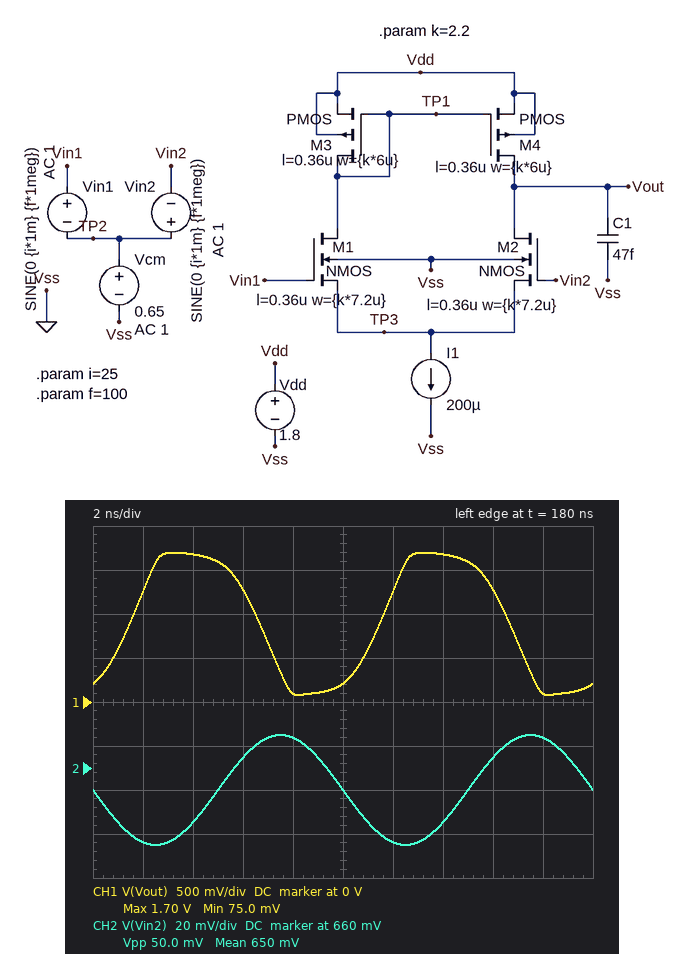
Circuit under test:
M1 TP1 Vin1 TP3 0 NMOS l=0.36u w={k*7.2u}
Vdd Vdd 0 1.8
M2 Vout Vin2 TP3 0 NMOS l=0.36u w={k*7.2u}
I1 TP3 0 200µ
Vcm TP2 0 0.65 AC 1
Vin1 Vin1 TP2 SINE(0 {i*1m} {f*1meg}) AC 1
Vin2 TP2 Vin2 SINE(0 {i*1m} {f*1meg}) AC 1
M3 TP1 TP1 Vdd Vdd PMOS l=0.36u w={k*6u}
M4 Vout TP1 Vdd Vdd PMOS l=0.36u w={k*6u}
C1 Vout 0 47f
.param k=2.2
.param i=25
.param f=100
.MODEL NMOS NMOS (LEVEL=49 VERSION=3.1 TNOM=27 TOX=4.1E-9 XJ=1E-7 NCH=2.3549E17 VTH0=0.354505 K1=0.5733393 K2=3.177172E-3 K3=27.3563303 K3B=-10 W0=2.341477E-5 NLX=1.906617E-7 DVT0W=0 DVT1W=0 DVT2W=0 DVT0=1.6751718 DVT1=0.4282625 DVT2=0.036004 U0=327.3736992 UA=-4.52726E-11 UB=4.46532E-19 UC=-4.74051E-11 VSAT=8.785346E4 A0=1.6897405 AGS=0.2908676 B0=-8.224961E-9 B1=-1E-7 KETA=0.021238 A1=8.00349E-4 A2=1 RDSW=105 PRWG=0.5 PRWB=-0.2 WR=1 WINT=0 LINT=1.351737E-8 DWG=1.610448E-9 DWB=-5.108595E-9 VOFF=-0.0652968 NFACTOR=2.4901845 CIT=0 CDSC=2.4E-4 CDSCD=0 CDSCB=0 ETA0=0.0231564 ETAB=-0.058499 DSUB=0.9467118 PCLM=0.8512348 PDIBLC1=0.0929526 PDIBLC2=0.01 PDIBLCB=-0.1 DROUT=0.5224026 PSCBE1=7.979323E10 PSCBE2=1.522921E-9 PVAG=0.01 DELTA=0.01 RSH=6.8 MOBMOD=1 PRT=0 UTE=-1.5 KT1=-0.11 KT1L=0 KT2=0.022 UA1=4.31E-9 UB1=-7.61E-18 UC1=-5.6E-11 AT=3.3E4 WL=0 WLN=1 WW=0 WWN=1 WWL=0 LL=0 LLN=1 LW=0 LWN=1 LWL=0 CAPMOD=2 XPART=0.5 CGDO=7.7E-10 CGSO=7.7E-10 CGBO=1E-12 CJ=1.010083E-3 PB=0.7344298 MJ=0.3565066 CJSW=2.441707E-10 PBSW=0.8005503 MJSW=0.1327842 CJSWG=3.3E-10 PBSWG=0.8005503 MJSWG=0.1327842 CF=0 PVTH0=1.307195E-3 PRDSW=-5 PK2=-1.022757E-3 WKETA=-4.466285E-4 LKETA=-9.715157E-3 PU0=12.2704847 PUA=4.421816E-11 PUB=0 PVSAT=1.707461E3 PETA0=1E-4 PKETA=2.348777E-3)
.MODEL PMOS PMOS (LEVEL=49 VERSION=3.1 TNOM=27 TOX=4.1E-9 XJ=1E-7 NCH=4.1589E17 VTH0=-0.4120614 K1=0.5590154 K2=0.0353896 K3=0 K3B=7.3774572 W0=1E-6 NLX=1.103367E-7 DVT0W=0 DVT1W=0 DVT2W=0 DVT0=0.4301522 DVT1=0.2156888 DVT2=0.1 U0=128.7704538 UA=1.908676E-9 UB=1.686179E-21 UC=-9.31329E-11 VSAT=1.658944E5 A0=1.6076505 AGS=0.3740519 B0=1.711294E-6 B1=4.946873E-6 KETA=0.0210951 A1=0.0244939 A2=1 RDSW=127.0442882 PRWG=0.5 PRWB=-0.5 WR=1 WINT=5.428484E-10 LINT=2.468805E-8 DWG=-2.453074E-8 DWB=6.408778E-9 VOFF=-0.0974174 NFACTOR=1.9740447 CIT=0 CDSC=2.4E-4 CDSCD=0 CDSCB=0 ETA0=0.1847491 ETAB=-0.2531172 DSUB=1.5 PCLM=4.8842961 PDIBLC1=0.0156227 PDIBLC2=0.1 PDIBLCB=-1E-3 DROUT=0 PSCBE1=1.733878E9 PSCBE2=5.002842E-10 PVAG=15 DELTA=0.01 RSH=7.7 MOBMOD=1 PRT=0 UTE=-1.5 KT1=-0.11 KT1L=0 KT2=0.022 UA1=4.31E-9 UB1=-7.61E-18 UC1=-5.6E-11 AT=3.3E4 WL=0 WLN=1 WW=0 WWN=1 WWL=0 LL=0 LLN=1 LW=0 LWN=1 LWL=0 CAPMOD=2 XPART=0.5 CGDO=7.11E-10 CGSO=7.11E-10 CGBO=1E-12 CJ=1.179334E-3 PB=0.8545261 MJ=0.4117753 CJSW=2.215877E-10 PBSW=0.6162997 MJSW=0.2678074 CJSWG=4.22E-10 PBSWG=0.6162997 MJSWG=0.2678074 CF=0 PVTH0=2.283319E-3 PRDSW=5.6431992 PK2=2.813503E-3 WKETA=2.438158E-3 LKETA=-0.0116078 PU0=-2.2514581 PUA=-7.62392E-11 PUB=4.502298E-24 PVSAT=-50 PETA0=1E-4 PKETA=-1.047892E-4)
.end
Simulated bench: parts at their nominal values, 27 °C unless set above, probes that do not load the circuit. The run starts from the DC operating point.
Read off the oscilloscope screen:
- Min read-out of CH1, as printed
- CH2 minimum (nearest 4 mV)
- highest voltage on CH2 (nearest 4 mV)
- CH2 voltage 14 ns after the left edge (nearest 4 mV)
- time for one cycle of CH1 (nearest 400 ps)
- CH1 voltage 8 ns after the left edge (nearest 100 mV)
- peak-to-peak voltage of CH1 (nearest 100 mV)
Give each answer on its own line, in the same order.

75.0 mV
624 mV
676 mV
636 mV
10.0 ns
100 mV
1.6 V
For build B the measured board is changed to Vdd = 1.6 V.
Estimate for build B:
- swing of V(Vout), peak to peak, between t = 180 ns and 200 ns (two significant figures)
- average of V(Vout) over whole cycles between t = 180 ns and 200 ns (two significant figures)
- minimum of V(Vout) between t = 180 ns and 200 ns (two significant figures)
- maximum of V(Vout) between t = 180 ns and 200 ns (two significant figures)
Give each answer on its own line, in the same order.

1.4 V
800 mV
69 mV
1.5 V
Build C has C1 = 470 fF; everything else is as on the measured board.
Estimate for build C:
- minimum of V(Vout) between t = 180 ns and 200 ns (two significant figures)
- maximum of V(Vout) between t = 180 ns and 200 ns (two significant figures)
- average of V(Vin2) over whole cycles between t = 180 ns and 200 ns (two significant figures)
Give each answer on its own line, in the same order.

830 mV
1.3 V
650 mV
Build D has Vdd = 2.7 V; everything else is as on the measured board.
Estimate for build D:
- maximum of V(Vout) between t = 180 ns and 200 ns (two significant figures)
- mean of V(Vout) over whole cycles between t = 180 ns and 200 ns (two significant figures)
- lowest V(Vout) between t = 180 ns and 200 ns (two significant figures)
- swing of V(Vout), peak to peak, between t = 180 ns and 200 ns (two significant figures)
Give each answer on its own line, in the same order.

2.6 V
1.6 V
470 mV
2.1 V
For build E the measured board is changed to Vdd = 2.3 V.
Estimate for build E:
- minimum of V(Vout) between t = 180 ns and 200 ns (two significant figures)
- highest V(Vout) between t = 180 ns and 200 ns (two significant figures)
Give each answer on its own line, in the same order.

150 mV
2.2 V
